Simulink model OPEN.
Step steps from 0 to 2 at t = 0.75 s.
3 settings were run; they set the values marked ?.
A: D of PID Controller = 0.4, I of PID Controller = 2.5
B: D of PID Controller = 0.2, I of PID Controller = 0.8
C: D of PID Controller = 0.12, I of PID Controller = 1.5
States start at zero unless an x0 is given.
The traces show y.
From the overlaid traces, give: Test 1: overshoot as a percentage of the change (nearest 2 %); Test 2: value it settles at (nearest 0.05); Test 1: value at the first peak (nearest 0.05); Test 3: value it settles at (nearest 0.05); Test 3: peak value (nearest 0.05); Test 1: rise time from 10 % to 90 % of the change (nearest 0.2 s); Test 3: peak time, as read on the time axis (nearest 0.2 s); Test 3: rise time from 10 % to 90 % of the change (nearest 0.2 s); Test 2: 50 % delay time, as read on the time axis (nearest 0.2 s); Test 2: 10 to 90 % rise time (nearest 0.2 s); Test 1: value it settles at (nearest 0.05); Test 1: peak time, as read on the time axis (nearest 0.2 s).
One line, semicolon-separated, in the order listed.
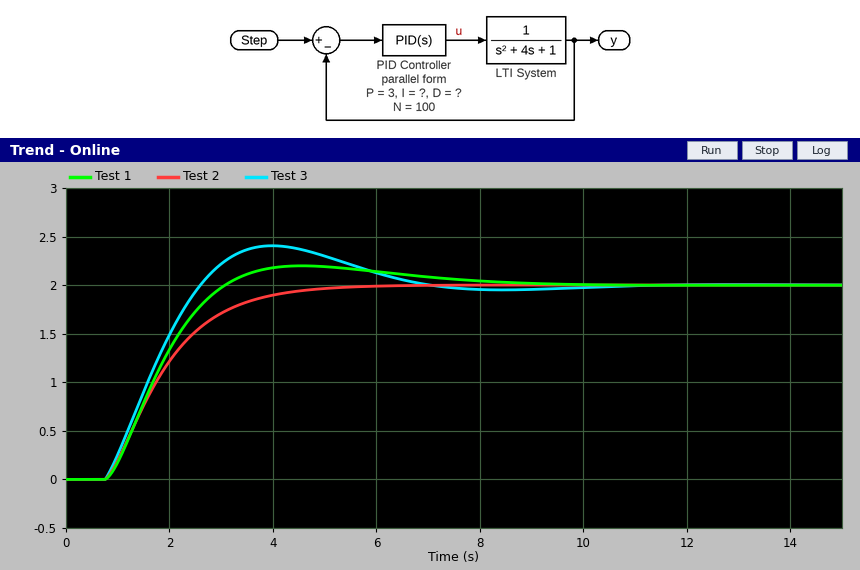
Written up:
10 %; 2.00; 2.20; 2.00; 2.40; 1.6 s; 4.0 s; 1.4 s; 1.8 s; 2.4 s; 2.00; 4.6 s
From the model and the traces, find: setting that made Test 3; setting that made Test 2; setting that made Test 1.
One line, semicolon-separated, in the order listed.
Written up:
A; B; C
